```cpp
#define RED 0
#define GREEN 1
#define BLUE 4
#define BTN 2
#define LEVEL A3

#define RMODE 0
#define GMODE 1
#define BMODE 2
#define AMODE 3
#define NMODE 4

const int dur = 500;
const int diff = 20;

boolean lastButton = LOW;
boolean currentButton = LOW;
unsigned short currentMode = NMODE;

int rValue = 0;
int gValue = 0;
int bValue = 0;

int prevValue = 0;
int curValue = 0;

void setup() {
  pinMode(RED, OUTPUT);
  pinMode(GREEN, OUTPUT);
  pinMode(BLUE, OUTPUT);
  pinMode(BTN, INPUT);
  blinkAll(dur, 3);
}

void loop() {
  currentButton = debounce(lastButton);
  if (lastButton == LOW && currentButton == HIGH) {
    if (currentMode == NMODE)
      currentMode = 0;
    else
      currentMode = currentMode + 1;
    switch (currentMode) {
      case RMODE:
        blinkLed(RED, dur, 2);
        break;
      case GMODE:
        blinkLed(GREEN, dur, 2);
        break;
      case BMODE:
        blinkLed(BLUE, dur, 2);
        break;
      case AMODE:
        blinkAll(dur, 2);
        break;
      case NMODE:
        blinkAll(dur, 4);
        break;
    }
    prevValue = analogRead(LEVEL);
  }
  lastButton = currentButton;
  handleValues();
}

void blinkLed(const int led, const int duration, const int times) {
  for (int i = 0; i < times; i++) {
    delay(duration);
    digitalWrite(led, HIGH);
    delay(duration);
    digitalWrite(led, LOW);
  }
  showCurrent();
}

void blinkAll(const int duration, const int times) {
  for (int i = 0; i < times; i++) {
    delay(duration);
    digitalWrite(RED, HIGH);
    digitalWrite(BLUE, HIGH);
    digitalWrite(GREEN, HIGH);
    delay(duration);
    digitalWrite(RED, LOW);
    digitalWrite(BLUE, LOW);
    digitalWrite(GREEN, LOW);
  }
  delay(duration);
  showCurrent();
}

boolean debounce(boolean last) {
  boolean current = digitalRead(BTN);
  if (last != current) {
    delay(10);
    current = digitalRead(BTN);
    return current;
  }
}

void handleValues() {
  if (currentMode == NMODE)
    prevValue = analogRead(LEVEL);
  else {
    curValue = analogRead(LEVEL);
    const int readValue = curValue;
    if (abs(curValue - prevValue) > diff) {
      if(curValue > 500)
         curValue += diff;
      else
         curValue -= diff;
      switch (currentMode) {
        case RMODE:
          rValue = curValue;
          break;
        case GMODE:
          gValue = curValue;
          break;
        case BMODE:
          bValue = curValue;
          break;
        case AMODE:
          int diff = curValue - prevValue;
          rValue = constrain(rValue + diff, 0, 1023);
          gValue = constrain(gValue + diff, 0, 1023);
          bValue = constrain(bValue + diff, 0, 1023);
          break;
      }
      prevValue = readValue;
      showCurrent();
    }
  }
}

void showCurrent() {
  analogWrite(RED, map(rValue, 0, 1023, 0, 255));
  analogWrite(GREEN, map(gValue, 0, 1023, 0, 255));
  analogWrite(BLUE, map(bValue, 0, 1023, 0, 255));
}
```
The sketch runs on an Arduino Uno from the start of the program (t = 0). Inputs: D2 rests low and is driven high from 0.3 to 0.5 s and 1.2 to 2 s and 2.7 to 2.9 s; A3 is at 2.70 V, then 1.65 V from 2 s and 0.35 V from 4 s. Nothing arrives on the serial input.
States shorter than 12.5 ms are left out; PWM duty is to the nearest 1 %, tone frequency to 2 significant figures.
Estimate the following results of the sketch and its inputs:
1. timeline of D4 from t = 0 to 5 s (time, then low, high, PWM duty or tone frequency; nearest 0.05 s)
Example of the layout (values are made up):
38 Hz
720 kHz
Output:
0 s low; 0.5 s high; 1 s low; 1.5 s high; 2 s low; 2.5 s high; 3 s low
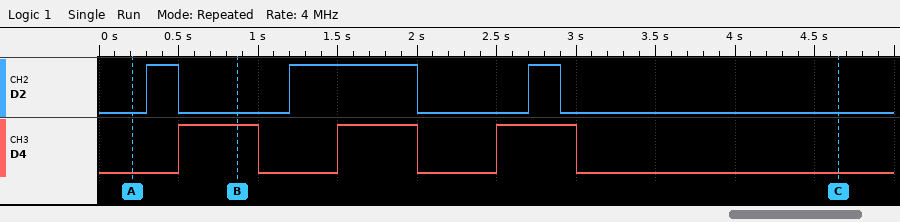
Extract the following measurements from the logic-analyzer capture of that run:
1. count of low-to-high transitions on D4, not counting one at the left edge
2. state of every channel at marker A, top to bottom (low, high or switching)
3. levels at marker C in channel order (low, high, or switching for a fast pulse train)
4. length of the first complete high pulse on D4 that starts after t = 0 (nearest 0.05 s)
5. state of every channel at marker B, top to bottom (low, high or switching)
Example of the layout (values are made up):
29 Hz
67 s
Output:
3
D2 low, D4 low
D2 low, D4 low
0.50 s
D2 low, D4 high
